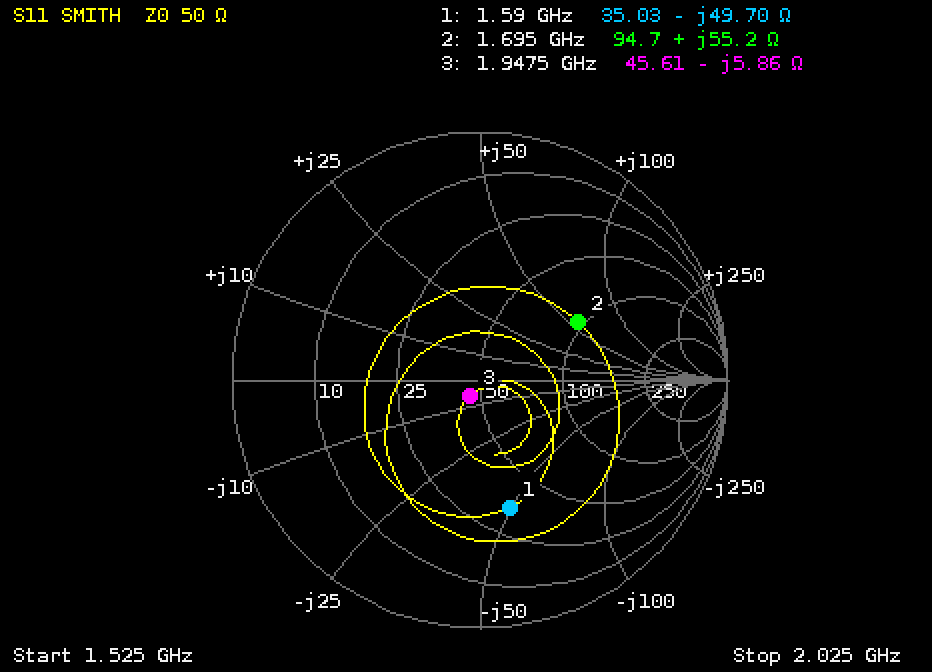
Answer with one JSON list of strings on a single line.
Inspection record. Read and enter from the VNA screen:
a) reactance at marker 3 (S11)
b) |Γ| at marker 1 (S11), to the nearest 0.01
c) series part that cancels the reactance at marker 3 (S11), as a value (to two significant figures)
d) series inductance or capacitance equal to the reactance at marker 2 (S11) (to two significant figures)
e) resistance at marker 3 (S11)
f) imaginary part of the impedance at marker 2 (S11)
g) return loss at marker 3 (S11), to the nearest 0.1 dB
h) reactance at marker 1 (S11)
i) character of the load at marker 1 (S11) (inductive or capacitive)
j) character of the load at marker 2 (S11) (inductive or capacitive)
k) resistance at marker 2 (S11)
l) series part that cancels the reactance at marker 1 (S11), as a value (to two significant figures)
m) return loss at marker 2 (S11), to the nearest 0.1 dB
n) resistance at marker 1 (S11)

["-5.86 Ω", "0.53", "480 pH", "5.2 nH", "45.61 Ω", "+55.2 Ω", "22.3 dB", "-49.70 Ω", "capacitive", "inductive", "94.7 Ω", "5.0 nH", "6.8 dB", "35.03 Ω"]
